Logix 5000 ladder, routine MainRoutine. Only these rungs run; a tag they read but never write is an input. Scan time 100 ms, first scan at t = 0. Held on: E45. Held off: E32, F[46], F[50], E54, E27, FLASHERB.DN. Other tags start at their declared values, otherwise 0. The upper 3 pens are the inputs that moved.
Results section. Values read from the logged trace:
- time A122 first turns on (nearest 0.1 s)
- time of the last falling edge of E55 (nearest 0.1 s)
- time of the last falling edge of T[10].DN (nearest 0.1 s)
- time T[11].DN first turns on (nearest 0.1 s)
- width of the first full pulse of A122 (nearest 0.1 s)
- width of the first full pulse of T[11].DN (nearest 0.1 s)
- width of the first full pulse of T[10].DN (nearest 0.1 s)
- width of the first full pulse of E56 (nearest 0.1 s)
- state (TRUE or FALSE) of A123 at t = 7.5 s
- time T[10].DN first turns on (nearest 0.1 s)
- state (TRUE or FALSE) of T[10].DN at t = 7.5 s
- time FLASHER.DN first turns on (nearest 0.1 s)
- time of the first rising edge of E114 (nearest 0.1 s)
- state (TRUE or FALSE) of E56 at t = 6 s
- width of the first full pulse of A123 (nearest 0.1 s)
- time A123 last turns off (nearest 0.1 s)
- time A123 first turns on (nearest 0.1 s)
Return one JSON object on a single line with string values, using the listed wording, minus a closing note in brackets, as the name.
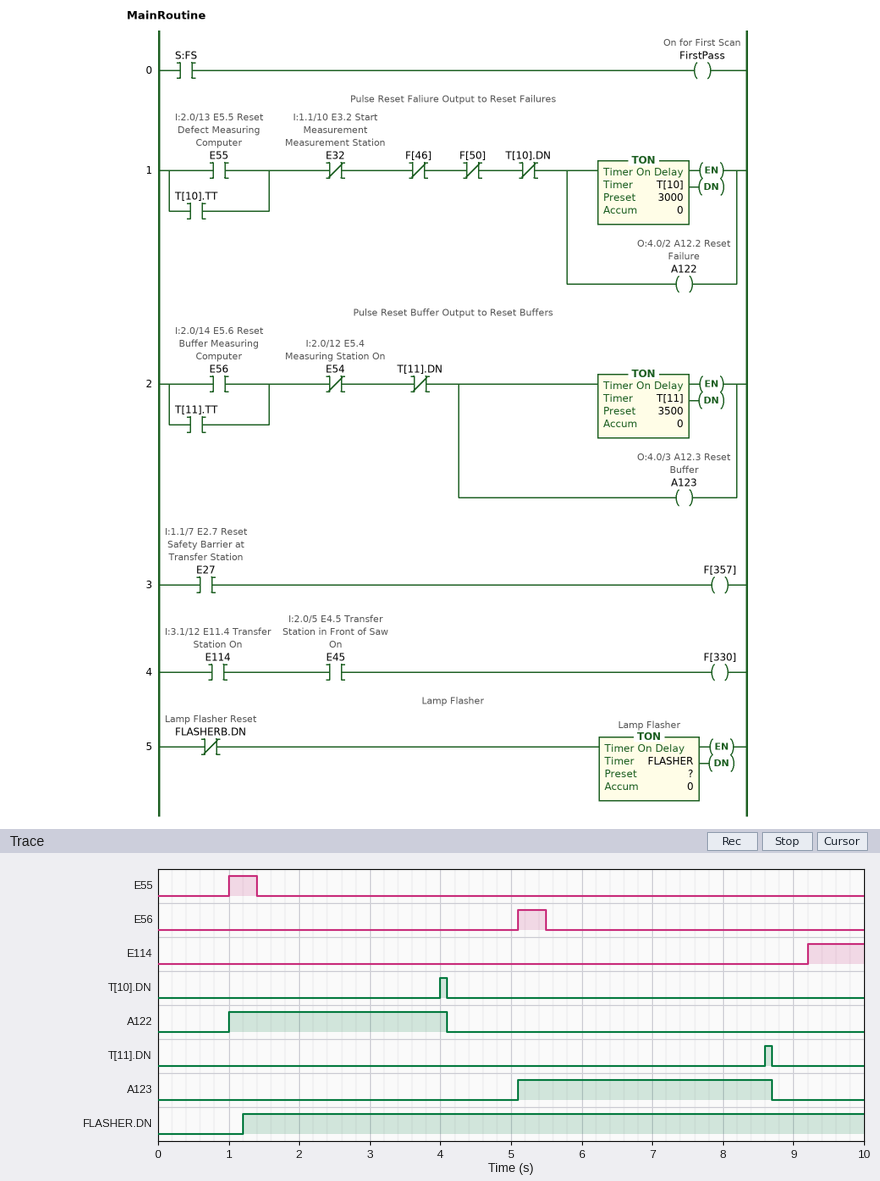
{"time A122 first turns on": "1.0 s", "time of the last falling edge of E55": "1.4 s", "time of the last falling edge of T[10].DN": "4.1 s", "time T[11].DN first turns on": "8.6 s", "width of the first full pulse of A122": "3.1 s", "width of the first full pulse of T[11].DN": "0.1 s", "width of the first full pulse of T[10].DN": "0.1 s", "width of the first full pulse of E56": "0.4 s", "state (TRUE or FALSE) of A123 at t = 7.5 s": "TRUE", "time T[10].DN first turns on": "4.0 s", "state (TRUE or FALSE) of T[10].DN at t = 7.5 s": "FALSE", "time FLASHER.DN first turns on": "1.2 s", "time of the first rising edge of E114": "9.2 s", "state (TRUE or FALSE) of E56 at t = 6 s": "FALSE", "width of the first full pulse of A123": "3.6 s", "time A123 last turns off": "8.7 s", "time A123 first turns on": "5.1 s"}
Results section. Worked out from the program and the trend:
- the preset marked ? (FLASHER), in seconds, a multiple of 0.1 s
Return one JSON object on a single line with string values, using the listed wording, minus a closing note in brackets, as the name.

{"the preset marked ? (FLASHER), in seconds, a multiple of 0.1 s": "1.2 s"}
